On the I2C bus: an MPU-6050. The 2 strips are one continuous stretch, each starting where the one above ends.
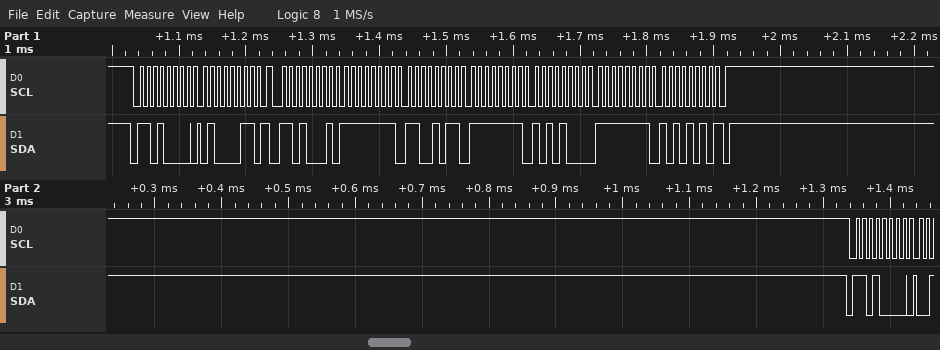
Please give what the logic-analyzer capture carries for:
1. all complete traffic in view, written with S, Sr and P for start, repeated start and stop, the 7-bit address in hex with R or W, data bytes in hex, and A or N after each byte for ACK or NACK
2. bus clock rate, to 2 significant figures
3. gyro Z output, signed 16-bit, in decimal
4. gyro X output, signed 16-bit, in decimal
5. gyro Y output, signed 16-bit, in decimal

S 68W A 43 A Sr 68R A FF A CB A FF A A8 A FF A AA N P S 68W A
100 kHz
-86
-53
-88
